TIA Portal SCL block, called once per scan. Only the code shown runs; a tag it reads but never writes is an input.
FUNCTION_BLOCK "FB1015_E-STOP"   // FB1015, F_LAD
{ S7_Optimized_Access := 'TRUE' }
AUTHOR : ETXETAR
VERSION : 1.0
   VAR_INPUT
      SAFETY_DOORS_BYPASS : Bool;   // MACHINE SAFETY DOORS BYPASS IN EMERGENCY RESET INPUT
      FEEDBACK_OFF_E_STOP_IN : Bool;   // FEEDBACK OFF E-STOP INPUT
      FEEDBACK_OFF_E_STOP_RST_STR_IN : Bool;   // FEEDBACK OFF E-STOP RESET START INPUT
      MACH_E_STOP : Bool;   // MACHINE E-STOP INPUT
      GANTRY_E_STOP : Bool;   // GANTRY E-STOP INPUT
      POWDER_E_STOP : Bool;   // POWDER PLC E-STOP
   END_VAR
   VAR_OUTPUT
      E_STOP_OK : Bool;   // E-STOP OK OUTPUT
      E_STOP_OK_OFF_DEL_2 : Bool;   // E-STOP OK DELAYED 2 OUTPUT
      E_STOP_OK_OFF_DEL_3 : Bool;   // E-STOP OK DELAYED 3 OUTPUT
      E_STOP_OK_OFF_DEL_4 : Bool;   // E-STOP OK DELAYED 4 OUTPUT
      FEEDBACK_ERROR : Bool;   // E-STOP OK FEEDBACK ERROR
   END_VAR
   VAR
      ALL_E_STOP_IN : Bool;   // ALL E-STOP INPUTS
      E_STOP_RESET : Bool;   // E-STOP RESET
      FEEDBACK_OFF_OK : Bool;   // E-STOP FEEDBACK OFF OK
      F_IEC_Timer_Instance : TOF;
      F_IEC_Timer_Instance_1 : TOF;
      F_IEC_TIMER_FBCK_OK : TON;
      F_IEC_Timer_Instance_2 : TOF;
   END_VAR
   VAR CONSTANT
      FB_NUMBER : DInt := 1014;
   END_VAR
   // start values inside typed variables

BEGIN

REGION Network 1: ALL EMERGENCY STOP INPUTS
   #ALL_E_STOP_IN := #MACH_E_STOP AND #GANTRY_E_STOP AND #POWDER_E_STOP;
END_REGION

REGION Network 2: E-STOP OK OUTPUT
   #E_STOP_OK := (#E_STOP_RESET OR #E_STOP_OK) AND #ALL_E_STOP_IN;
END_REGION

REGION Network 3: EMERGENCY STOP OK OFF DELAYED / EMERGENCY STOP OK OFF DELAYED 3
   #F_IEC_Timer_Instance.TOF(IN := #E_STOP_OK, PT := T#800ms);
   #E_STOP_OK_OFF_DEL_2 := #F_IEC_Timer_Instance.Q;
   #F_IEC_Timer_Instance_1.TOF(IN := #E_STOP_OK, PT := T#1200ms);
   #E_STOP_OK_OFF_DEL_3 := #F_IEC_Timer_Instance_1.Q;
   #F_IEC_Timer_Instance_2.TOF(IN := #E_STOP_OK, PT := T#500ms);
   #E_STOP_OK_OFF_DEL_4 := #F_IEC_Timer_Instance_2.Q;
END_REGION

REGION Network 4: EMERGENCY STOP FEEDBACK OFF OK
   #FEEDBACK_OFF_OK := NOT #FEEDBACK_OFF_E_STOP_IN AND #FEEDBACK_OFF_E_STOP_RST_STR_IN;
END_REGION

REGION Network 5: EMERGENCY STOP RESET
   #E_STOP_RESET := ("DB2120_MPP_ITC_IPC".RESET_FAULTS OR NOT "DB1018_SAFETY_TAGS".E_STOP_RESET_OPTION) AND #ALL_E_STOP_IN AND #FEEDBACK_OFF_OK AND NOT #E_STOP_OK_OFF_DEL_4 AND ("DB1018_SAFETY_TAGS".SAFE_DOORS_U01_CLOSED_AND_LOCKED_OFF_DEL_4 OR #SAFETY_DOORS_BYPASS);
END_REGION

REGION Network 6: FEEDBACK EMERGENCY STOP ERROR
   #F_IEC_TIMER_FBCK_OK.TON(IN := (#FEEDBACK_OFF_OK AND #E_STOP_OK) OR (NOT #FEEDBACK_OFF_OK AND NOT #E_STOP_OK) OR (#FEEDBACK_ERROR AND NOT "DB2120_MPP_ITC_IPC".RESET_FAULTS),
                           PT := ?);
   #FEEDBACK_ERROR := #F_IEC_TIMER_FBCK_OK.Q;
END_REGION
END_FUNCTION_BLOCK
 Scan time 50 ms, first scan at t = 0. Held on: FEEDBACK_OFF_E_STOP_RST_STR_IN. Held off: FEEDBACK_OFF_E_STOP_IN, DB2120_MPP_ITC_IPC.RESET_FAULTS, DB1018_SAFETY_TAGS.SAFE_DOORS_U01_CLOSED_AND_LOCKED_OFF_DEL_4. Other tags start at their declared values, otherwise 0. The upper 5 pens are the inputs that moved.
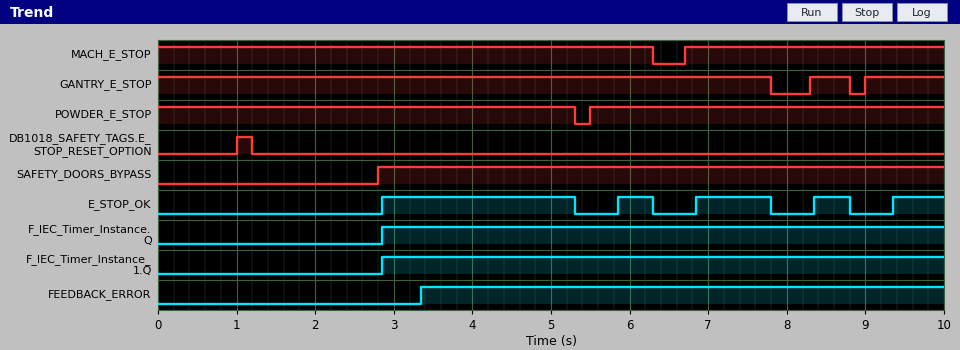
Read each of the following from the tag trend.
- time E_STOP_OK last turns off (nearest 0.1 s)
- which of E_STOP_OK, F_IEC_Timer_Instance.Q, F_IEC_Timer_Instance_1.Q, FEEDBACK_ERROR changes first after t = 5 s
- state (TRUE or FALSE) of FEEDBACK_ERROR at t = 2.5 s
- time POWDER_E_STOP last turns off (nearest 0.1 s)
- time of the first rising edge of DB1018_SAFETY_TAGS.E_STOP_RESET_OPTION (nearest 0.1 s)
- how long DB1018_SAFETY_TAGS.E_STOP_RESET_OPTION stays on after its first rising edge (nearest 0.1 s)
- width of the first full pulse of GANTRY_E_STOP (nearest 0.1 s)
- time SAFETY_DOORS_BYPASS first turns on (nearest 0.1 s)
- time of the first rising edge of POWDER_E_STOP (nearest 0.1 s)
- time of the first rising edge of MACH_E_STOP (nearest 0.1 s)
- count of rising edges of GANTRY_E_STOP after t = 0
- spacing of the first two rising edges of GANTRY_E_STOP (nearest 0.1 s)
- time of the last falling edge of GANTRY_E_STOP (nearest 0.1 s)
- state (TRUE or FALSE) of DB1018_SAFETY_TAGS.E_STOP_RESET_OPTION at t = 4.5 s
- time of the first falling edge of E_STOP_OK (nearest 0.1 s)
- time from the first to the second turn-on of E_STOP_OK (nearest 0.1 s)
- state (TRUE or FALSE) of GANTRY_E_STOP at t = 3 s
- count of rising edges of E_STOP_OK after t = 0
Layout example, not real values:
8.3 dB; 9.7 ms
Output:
8.8 s; E_STOP_OK; FALSE; 5.3 s; 1.0 s; 0.2 s; 0.5 s; 2.8 s; 5.5 s; 6.7 s; 2; 0.7 s; 8.8 s; FALSE; 5.3 s; 3.0 s; TRUE; 5
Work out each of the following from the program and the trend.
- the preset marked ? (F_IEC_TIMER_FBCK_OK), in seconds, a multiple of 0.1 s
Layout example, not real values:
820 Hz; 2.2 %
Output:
0.5 s
